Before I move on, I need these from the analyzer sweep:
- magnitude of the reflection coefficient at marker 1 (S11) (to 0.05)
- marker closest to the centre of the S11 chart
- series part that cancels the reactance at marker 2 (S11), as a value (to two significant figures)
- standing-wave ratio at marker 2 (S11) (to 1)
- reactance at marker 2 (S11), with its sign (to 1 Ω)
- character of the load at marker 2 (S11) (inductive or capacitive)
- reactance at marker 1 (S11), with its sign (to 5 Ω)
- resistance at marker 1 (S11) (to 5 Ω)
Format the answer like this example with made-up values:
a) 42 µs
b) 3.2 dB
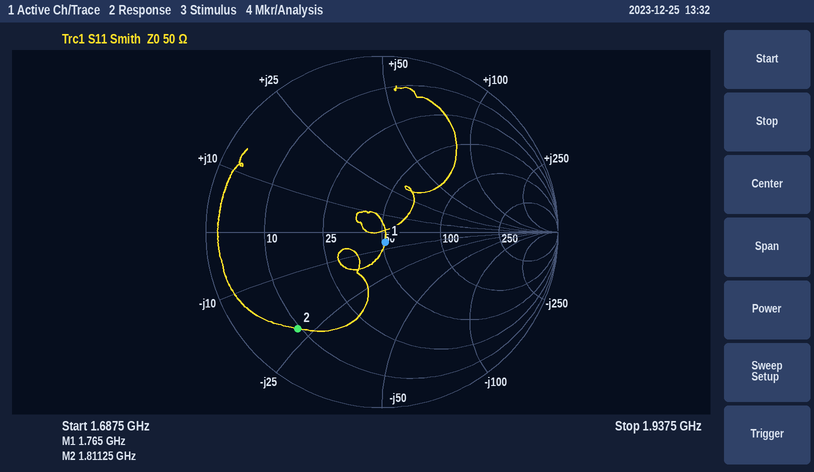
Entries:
a) 0.05
b) marker 1
c) 1.9 nH
d) 6
e) -22 Ω
f) capacitive
g) -5 Ω
h) 50 Ω
